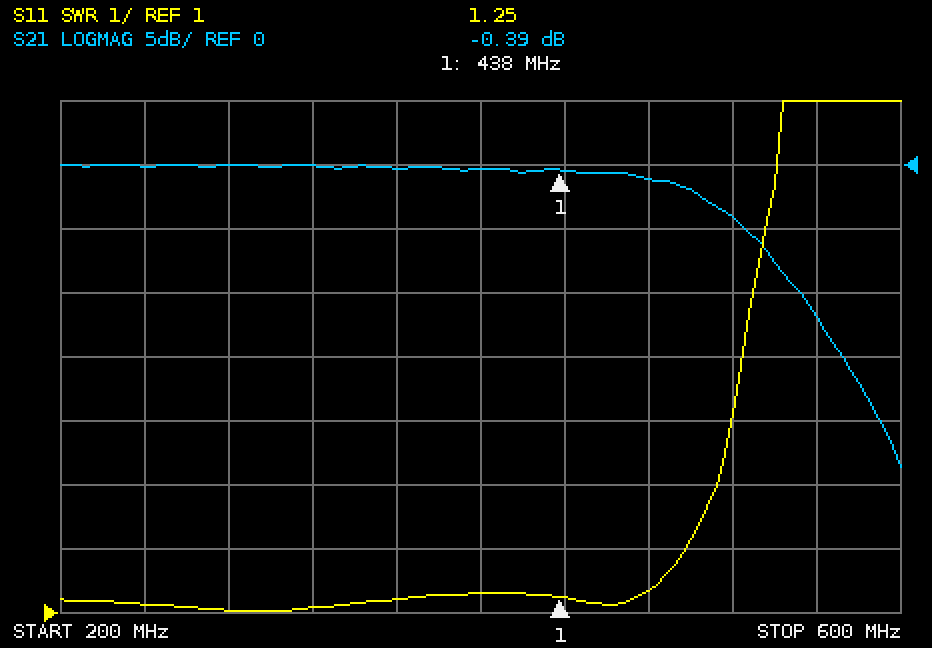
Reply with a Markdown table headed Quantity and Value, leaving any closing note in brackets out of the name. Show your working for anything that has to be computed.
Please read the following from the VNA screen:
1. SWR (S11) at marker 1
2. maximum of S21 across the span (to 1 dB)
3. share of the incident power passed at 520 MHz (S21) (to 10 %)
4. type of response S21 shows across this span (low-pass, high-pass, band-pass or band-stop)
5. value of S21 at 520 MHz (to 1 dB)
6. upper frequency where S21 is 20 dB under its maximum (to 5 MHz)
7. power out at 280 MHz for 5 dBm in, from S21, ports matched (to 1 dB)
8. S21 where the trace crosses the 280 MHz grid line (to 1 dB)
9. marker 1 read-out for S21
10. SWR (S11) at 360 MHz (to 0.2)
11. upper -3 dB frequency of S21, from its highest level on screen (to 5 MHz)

| Quantity | Value |
|---|---|
| SWR (S11) at marker 1 | 1.25 |
| maximum of S21 across the span | 0 dB |
| share of the incident power passed at 520 MHz (S21) | 10^(-4/10) ≈ 40 % |
| type of response S21 shows across this span | low-pass |
| value of S21 at 520 MHz | -4 dB |
| upper frequency where S21 is 20 dB under its maximum | 590 MHz |
| power out at 280 MHz for 5 dBm in, from S21, ports matched | 5 dBm + (0 dB) = 5 dBm |
| S21 where the trace crosses the 280 MHz grid line | 0 dB |
| marker 1 read-out for S21 | -0.39 dB |
| SWR (S11) at 360 MHz | 1.2 |
| upper -3 dB frequency of S21, from its highest level on screen | 510 MHz |
